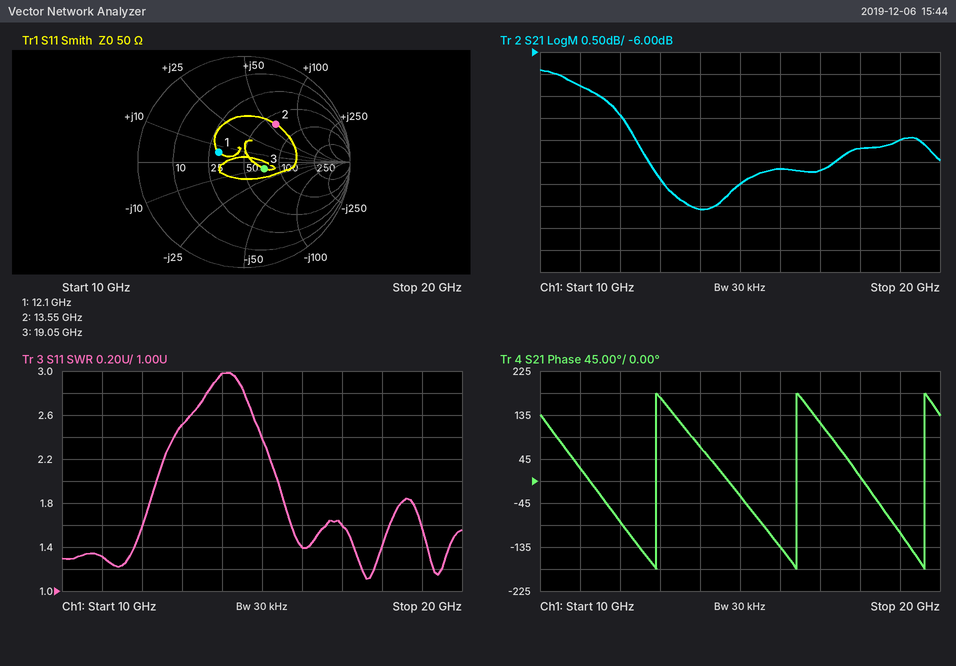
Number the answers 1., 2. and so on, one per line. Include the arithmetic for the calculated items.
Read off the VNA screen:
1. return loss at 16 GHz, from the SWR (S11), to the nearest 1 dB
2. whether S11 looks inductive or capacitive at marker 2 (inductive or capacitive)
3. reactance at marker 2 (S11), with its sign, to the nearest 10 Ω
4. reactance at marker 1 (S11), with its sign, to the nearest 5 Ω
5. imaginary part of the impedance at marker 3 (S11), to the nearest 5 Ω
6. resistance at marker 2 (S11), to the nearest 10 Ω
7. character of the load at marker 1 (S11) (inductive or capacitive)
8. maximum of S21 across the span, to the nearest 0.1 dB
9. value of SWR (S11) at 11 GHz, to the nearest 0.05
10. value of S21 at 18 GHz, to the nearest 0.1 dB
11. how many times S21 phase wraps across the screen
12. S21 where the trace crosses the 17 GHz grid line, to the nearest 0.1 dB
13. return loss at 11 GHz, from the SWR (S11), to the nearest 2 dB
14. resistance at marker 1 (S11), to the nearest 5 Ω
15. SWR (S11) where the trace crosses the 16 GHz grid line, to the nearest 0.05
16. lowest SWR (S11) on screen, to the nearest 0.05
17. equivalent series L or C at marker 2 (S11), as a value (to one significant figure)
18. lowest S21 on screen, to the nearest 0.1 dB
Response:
1. −20 log10((1.4 − 1)/(1.4 + 1)) ≈ 16 dB
2. inductive
3. +60 Ω
4. +5 Ω
5. -10 Ω
6. 60 Ω
7. inductive
8. -6.4 dB
9. 1.30
10. -8.2 dB
11. 3
12. -8.7 dB
13. −20 log10((1.3 − 1)/(1.3 + 1)) ≈ 18 dB
14. 30 Ω
15. 1.40
16. 1.10
17. L = 60 Ω/(2π × 13.55 GHz) ≈ 705 pH, so 700 pH to one significant figure
18. -9.6 dB
